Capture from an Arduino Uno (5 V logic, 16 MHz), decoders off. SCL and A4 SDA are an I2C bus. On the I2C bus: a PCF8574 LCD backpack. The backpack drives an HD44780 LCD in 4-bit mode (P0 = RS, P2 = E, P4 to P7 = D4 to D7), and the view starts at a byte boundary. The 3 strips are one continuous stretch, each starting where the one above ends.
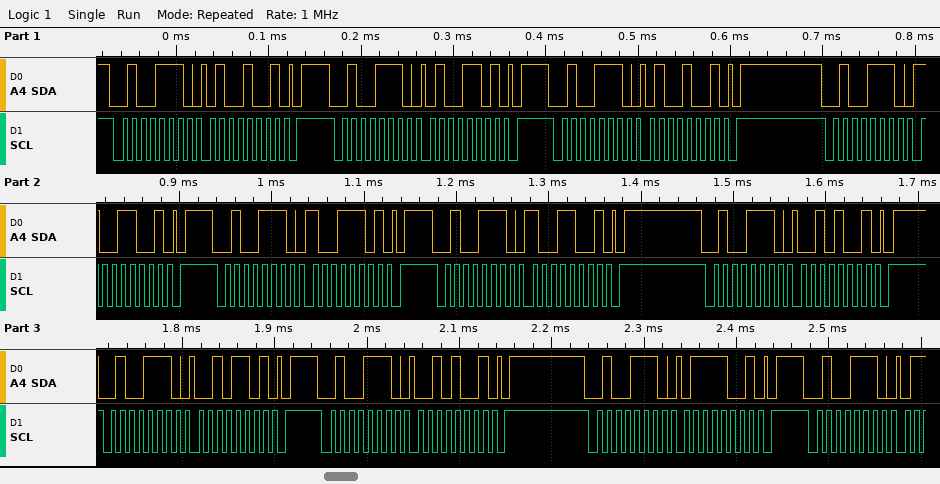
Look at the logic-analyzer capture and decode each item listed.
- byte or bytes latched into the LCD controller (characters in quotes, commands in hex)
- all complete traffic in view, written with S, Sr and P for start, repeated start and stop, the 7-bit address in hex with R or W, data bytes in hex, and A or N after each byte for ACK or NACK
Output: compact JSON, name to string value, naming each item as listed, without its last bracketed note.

{"byte or bytes latched into the LCD controller": "'I'", "all complete traffic in view, written with S, Sr and P for start, repeated start and stop, the 7-bit address in hex with R or W, data bytes in hex, and A or N after each byte for ACK or NACK": "S 27W A 49 A P S 27W A 4D A P S 27W A 49 A P S 27W A 99 A P S 27W A 9D A P S 27W A 99 A P S 27W A 29 A P S 27W A 2D A P S 27W A 29 A P S 27W A 79 A P S 27W A"}
